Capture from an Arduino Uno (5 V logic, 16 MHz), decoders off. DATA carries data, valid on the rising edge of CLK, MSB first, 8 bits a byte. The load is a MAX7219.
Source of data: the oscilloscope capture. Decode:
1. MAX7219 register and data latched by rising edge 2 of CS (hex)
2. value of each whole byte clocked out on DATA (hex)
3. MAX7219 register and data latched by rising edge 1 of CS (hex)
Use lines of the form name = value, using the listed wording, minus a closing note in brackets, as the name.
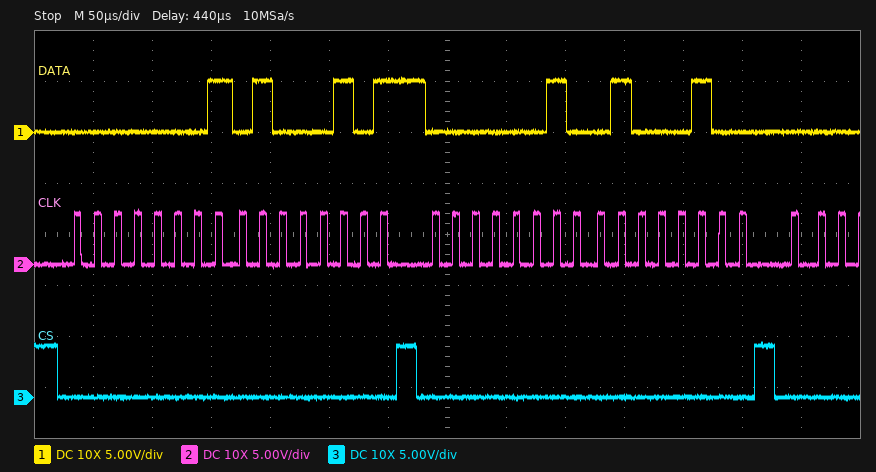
MAX7219 register and data latched by rising edge 2 of CS = register 0x2, data 0x44
value of each whole byte clocked out on DATA = 01 45 02 44
MAX7219 register and data latched by rising edge 1 of CS = register 0x1, data 0x45
